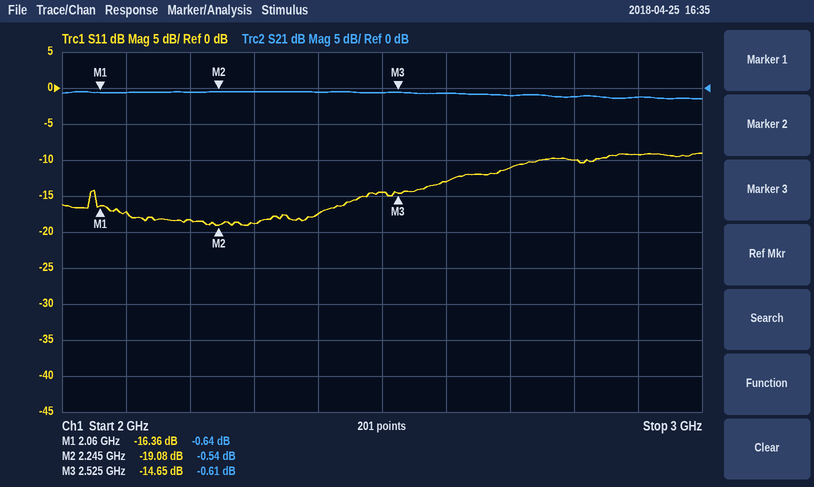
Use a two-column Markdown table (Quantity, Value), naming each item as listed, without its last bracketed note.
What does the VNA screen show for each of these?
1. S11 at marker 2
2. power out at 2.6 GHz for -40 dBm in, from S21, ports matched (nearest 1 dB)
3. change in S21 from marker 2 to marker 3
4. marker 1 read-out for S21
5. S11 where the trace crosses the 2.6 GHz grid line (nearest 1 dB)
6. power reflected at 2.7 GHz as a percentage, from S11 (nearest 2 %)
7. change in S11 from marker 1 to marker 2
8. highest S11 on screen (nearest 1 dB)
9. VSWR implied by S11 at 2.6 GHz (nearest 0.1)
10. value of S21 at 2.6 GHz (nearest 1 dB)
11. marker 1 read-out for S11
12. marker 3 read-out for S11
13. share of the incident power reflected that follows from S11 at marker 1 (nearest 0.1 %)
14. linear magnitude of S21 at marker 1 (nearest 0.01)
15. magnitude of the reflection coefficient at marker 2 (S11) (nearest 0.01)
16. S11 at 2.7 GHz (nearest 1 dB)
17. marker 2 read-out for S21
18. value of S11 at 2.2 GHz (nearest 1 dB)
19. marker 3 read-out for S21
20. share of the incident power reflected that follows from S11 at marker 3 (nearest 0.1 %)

| Quantity | Value |
|---|---|
| S11 at marker 2 | -19.08 dB |
| power out at 2.6 GHz for -40 dBm in, from S21, ports matched | -41 dBm |
| change in S21 from marker 2 to marker 3 | -0.07 dB |
| marker 1 read-out for S21 | -0.64 dB |
| S11 where the trace crosses the 2.6 GHz grid line | -13 dB |
| power reflected at 2.7 GHz as a percentage, from S11 | 8 % |
| change in S11 from marker 1 to marker 2 | -2.72 dB |
| highest S11 on screen | -9 dB |
| VSWR implied by S11 at 2.6 GHz | 1.6 |
| value of S21 at 2.6 GHz | -1 dB |
| marker 1 read-out for S11 | -16.36 dB |
| marker 3 read-out for S11 | -14.65 dB |
| share of the incident power reflected that follows from S11 at marker 1 | 2.3 % |
| linear magnitude of S21 at marker 1 | 0.93 |
| magnitude of the reflection coefficient at marker 2 (S11) | 0.11 |
| S11 at 2.7 GHz | -11 dB |
| marker 2 read-out for S21 | -0.54 dB |
| value of S11 at 2.2 GHz | -18 dB |
| marker 3 read-out for S21 | -0.61 dB |
| share of the incident power reflected that follows from S11 at marker 3 | 3.4 % |
